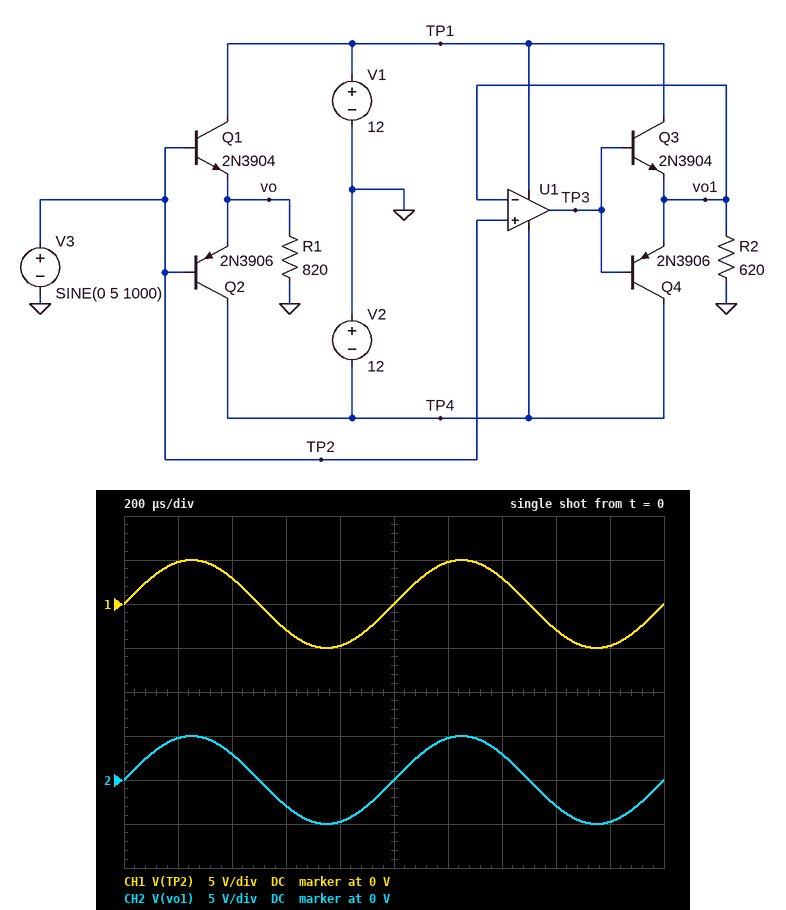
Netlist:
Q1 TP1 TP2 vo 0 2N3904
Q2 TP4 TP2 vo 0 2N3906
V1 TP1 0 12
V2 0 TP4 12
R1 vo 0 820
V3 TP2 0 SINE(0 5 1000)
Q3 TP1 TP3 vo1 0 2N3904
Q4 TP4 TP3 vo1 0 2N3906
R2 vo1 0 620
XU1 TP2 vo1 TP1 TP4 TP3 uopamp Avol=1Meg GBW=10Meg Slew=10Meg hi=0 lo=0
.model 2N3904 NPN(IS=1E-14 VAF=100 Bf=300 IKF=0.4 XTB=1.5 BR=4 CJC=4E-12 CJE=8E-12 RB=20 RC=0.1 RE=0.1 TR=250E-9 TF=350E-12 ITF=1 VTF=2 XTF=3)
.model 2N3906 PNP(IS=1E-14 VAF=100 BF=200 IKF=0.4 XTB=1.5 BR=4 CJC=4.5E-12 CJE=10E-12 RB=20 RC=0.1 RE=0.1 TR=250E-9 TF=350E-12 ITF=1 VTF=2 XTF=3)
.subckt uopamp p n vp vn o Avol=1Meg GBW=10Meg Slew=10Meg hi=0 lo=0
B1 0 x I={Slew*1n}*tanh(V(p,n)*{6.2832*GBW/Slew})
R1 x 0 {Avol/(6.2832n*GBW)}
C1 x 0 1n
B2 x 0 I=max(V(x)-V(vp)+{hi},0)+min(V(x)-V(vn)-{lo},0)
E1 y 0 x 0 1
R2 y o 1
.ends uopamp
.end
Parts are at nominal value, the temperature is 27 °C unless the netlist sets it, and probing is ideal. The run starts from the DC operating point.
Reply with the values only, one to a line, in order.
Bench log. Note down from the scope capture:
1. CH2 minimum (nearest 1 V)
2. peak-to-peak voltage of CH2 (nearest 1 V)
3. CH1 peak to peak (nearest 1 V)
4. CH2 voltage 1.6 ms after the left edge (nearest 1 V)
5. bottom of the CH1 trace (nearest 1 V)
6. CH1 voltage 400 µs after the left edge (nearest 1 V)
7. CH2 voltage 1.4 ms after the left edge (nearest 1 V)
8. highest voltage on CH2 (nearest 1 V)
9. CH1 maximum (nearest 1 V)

-5 V
10 V
10 V
-3 V
-5 V
3 V
3 V
5 V
5 V
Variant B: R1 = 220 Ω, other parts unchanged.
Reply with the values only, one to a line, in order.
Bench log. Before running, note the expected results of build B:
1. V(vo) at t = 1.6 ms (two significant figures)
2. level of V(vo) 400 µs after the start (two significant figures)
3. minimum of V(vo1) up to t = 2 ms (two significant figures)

-2.2 V
2.2 V
-5.0 V
